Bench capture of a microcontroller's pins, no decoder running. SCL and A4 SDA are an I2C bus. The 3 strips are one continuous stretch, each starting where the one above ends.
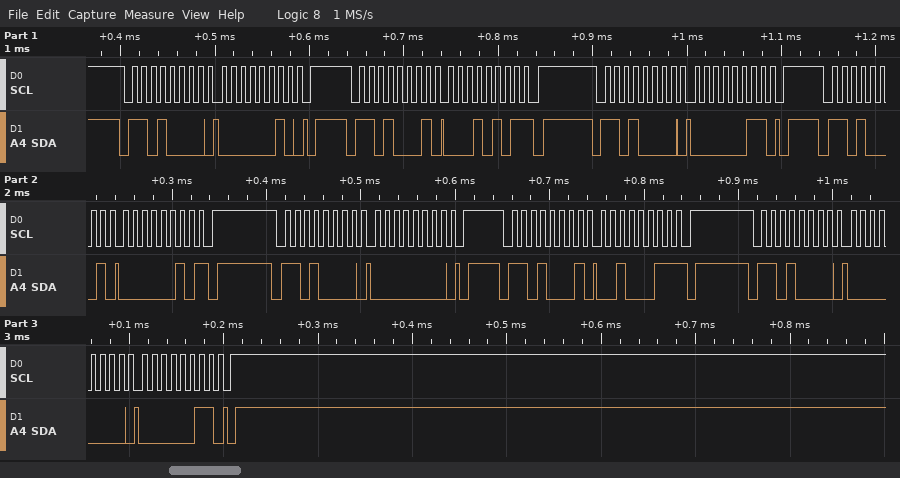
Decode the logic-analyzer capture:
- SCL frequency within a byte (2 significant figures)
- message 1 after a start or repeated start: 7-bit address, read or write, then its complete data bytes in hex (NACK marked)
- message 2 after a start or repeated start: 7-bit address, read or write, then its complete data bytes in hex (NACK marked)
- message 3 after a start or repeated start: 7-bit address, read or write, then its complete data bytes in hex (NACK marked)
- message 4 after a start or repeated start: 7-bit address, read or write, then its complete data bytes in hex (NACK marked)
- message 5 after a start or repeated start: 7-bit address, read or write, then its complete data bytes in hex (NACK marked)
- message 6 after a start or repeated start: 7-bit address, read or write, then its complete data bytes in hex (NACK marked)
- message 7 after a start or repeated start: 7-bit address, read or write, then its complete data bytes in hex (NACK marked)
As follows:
100 kHz
0x68 write: 02
0x68 read: 15 NACK
0x68 write: 03
0x68 read: 02 NACK
0x68 write: 00
0x68 read: 23 NACK
0x68 write: 00 03
